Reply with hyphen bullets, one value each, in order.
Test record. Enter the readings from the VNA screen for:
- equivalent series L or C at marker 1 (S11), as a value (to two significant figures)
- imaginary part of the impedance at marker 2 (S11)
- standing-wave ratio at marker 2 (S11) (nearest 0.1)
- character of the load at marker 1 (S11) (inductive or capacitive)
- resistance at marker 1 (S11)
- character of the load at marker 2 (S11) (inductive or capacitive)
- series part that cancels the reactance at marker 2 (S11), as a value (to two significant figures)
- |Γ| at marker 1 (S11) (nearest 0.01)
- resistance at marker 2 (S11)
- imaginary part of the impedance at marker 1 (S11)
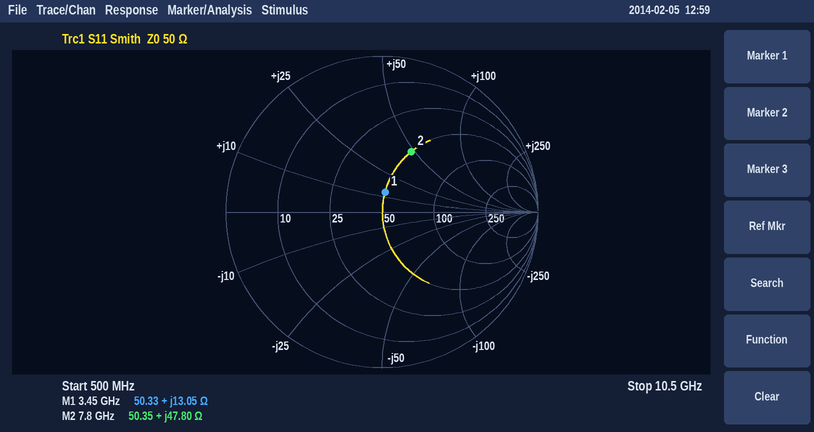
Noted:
- 600 pH
- +47.80 Ω
- 2.5
- inductive
- 50.33 Ω
- inductive
- 430 fF
- 0.13
- 50.35 Ω
- +13.05 Ω
